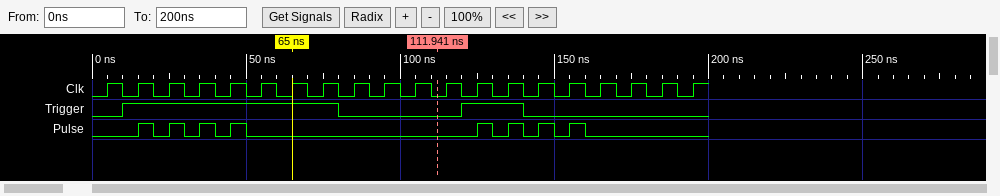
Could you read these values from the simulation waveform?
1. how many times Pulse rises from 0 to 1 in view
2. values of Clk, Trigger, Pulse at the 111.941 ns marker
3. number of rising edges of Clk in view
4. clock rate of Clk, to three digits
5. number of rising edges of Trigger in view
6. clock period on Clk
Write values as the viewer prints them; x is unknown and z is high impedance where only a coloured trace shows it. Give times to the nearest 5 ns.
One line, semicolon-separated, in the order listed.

8; Clk=0, Trigger=0, Pulse=0; 20; 100 MHz; 2; 10 ns
